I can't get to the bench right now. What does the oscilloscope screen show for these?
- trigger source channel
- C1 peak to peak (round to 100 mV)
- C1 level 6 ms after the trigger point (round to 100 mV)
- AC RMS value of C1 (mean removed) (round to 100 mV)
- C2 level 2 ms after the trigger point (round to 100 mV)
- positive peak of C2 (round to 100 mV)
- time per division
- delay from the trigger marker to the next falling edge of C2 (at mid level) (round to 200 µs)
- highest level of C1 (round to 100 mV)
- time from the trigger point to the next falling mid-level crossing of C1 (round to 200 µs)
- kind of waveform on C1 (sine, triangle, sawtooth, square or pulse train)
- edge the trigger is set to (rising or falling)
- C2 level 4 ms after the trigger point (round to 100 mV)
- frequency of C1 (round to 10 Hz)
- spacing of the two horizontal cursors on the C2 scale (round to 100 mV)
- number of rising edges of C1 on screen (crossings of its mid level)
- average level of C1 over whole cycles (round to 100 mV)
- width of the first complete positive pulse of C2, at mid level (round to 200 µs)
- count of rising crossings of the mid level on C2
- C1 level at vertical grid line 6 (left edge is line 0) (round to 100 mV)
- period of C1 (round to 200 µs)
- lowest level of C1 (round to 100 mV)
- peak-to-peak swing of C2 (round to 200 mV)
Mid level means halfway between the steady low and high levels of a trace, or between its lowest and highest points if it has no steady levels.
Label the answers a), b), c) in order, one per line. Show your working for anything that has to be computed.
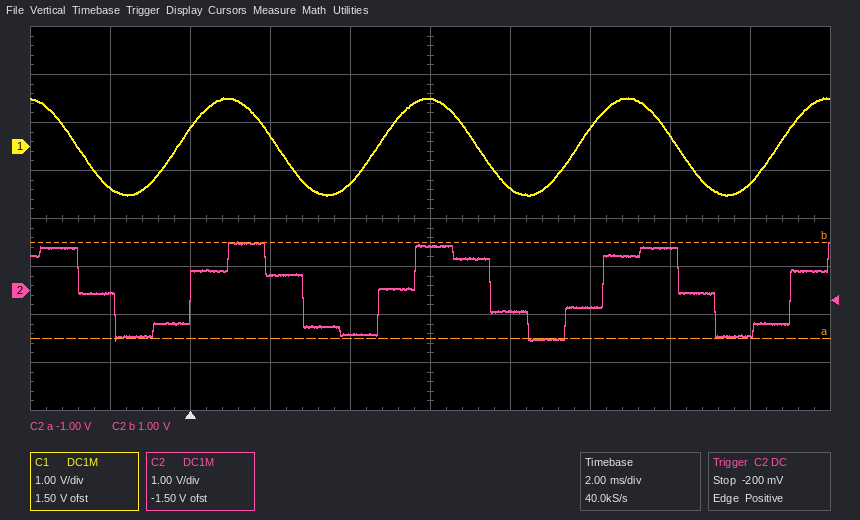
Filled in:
a) C2
b) 1.0 V − (-1.0 V) = 2.0 V
c) 1.0 V
d) 2.0 V / (2√2) ≈ 707 mV, so 700 mV to the nearest 100 mV
e) 300 mV
f) 1.0 V
g) 2 ms
h) 2.8 ms
i) 1.0 V
j) 2.2 ms
k) sine
l) rising
m) -900 mV
n) 1 / 5.0 ms ≈ 200 Hz
o) 2.0 V
p) 4
q) (1.0 V + (-1.0 V)) / 2 ≈ 0.0 V
r) 2.8 ms
s) 4
t) -900 mV
u) 5.0 ms
v) -1.0 V
w) 2.0 V
